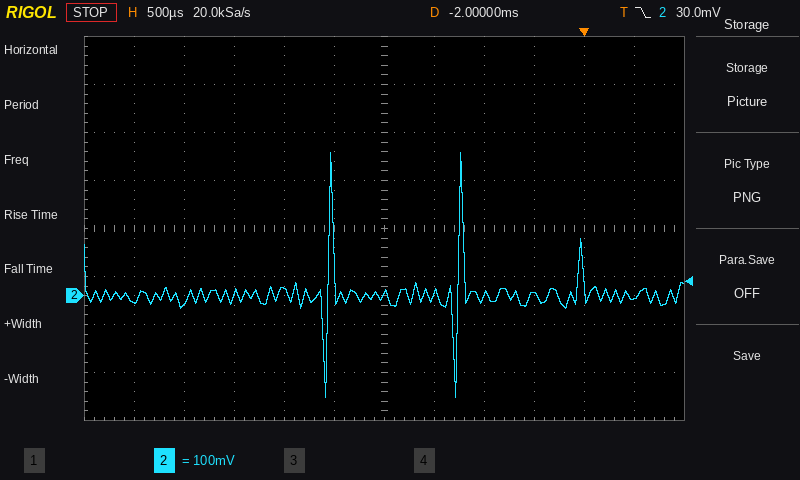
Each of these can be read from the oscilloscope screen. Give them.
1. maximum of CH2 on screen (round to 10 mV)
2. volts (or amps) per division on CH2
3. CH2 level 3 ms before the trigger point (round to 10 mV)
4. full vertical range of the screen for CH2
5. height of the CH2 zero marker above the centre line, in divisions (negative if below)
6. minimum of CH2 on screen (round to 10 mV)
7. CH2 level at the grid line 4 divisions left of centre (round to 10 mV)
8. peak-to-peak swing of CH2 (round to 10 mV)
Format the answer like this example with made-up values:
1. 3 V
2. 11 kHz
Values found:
1. 300 mV
2. 100 mV
3. 10 mV
4. 800 mV
5. -1.4 div
6. -210 mV
7. -20 mV
8. 510 mV
